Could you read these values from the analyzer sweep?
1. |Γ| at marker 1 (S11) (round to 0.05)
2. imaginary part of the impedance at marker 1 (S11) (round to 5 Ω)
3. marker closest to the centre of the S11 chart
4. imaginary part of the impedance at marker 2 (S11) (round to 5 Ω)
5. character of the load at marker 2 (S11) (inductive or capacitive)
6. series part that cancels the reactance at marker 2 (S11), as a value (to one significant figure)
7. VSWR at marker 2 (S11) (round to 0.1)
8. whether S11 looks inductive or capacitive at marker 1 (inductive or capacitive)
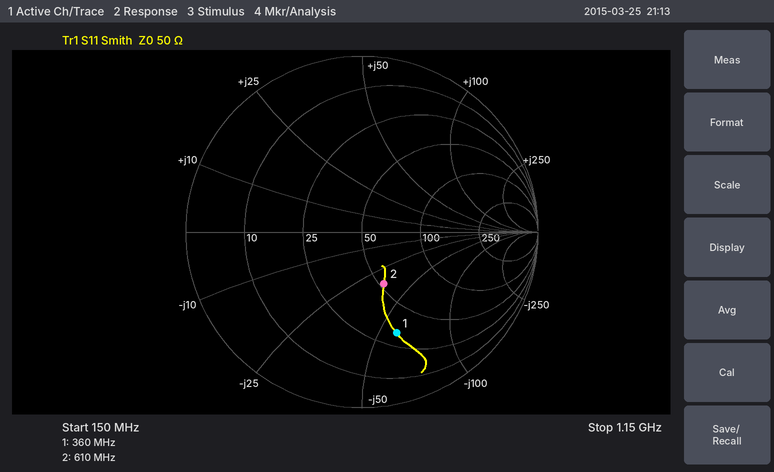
0.60
-60 Ω
marker 2
-35 Ω
capacitive
9 nH
1.9
capacitive
